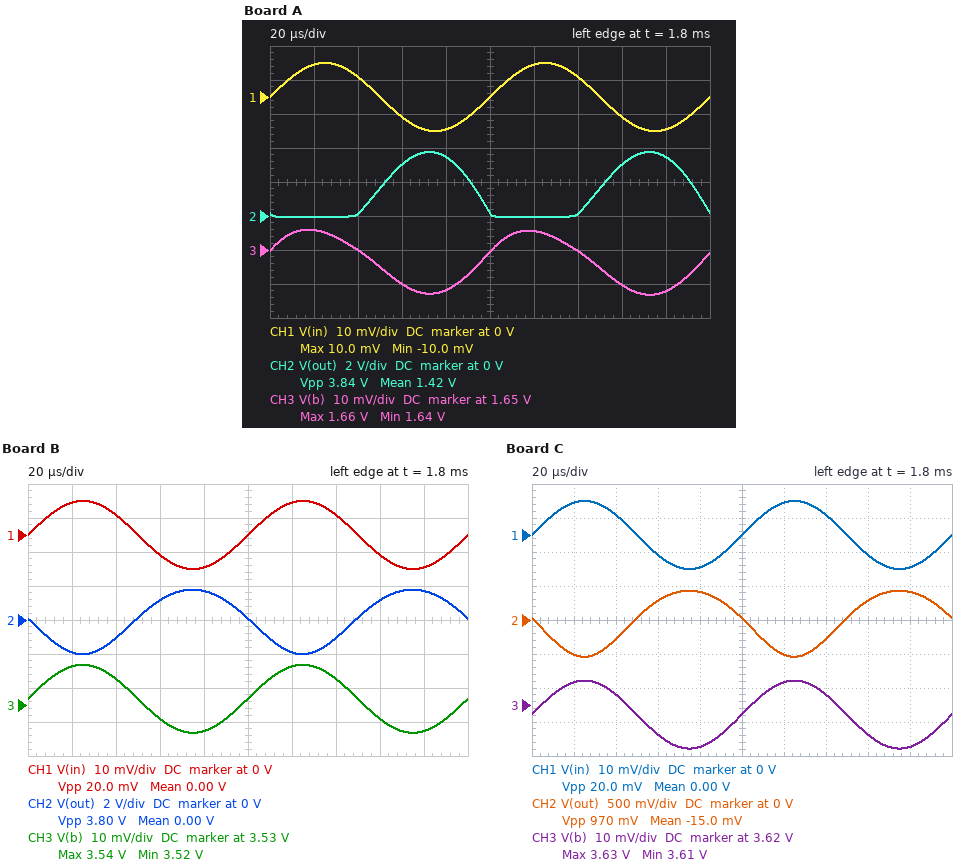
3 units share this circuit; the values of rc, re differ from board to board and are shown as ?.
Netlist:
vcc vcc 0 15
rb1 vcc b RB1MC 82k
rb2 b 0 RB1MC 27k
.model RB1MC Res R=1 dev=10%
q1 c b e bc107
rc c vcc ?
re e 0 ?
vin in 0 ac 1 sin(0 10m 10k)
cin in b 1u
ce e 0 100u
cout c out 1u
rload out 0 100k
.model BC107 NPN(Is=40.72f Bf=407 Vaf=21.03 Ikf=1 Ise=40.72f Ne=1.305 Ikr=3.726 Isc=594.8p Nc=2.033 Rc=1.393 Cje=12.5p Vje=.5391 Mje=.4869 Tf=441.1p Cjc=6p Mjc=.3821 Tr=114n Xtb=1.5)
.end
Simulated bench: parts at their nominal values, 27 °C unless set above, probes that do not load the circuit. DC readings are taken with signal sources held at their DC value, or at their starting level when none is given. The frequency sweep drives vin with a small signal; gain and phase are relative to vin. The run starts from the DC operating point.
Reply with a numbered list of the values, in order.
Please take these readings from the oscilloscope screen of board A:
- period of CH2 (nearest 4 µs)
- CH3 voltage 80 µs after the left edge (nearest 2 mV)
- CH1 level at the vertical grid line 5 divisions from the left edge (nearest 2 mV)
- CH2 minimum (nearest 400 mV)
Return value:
1. 100 µs
2. 1.638 V
3. 0 V
4. 0 V
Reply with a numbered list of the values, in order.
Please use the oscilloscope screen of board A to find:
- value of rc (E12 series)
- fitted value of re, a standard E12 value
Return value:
1. 4.7 kΩ
2. 330 Ω
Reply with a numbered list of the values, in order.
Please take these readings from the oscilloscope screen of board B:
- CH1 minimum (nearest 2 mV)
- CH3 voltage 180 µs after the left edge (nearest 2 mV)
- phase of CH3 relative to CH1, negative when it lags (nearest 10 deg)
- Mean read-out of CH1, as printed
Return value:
1. -10 mV
2. 3.522 V
3. 0 deg
4. 0.00 V
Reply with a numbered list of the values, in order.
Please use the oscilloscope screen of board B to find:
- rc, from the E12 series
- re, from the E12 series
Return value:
1. 3.3 kΩ
2. 1.5 kΩ
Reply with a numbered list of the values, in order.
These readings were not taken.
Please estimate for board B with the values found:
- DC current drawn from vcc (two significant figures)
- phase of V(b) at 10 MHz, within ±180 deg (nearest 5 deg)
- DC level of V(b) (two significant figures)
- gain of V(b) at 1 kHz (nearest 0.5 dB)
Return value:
1. 2.1 mA
2. 0 deg
3. 3.5 V
4. 0 dB
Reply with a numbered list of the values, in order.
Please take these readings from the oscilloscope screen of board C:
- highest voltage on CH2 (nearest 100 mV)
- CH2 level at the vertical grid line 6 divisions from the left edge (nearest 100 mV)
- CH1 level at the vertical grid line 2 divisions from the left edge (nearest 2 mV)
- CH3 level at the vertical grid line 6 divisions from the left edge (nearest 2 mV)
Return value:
1. 400 mV
2. -500 mV
3. 6 mV
4. 3.626 V
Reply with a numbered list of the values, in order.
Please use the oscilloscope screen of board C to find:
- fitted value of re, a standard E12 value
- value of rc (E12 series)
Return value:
1. 2.7 kΩ
2. 1.2 kΩ
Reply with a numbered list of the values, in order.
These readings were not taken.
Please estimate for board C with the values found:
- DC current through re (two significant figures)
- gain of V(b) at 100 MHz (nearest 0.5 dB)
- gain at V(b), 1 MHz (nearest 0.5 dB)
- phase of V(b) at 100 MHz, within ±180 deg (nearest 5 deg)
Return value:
1. 1.1 mA
2. 0 dB
3. 0 dB
4. 0 deg
